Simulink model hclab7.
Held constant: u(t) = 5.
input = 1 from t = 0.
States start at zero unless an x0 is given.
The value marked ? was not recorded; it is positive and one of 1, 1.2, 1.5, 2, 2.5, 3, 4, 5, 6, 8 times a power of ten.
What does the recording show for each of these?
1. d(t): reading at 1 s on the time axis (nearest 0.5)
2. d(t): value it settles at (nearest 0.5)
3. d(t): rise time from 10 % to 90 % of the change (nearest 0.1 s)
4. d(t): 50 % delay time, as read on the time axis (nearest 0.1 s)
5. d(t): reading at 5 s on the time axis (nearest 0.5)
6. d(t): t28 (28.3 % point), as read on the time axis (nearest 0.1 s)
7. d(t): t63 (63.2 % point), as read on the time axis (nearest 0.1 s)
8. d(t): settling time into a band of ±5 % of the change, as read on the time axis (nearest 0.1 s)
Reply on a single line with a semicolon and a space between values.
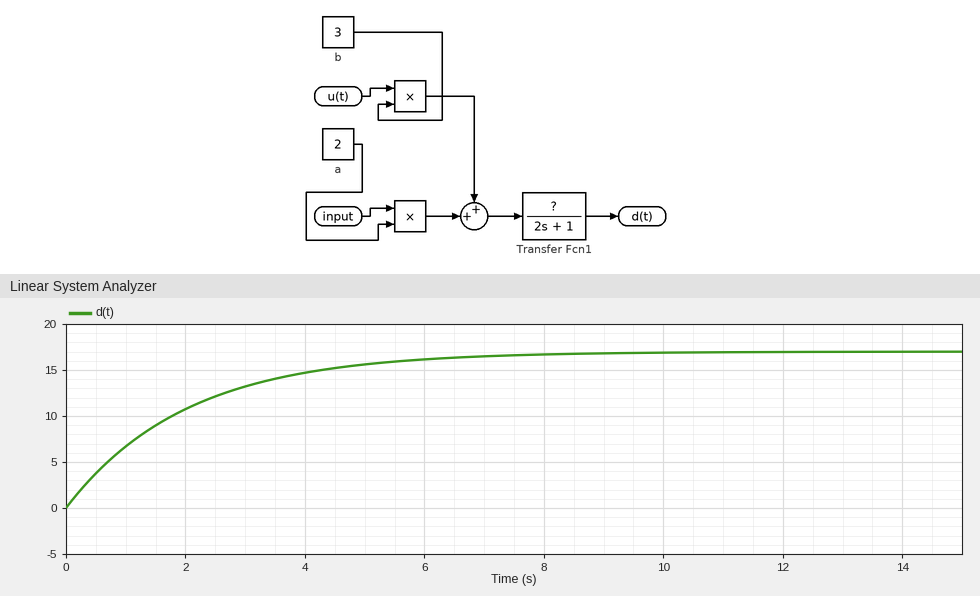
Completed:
6.5; 17.0; 4.4 s; 1.4 s; 15.5; 0.7 s; 2.0 s; 6.0 s
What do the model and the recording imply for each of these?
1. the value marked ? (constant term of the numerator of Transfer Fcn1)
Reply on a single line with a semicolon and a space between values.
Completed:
1
